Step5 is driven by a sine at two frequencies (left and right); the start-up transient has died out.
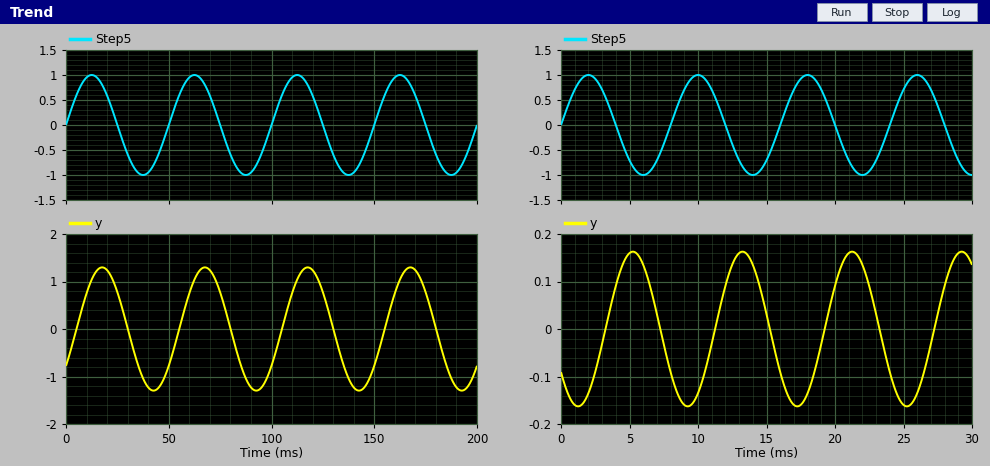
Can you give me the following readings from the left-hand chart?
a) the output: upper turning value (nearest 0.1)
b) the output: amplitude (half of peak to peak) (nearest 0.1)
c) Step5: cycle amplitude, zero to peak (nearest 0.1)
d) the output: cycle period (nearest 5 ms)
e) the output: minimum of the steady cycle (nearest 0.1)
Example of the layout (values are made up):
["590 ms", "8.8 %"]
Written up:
["1.3", "1.3", "1.0", "50 ms", "-1.3"]
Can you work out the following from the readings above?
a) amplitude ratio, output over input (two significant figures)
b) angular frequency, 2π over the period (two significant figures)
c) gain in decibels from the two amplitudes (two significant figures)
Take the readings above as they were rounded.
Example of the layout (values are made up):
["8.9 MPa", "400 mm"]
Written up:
["1.3", "0.13 rad/ms", "2.3 dB"]
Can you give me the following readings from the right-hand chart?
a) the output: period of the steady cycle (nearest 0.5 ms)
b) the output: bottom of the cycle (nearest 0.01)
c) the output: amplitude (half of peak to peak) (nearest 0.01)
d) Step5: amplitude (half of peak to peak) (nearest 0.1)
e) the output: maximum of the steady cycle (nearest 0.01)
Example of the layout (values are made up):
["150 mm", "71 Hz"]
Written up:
["8.0 ms", "-0.16", "0.16", "1.0", "0.16"]
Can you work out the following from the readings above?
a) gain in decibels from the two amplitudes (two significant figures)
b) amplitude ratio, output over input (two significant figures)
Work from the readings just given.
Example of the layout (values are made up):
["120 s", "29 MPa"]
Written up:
["-16 dB", "0.16"]
